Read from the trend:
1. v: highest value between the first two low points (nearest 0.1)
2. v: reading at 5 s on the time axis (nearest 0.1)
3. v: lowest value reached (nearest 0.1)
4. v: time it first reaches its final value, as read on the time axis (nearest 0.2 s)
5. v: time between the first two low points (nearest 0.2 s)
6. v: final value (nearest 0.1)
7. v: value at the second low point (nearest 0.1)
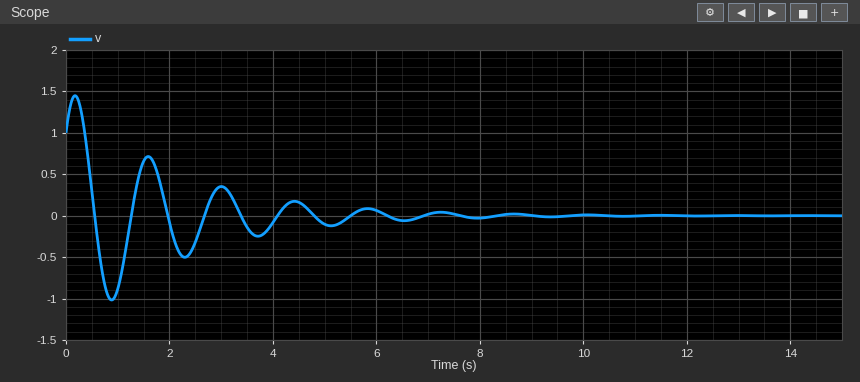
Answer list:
0.7
-0.1
-1.0
0.6 s
1.4 s
0.0
-0.5
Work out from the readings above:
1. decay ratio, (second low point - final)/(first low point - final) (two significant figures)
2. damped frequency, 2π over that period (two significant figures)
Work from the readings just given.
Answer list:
0.50
4.5 rad/s
